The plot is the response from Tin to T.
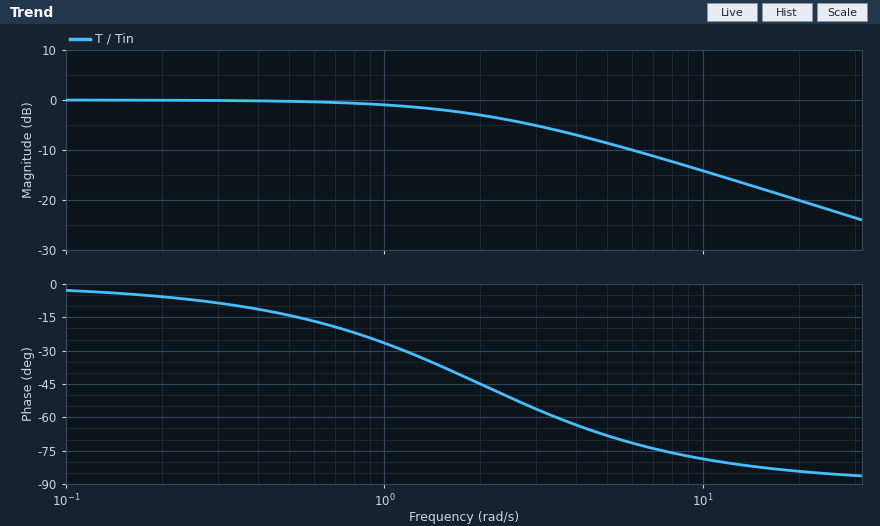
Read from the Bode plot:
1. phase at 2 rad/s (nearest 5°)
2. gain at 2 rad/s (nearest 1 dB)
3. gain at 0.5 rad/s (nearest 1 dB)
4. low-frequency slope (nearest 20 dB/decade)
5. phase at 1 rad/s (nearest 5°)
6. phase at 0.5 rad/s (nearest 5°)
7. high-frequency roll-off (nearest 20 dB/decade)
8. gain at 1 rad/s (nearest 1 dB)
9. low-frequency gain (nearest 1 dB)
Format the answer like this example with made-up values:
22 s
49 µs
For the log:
-45°
-3 dB
0 dB
0 dB/decade
-25°
-15°
-20 dB/decade
-1 dB
0 dB
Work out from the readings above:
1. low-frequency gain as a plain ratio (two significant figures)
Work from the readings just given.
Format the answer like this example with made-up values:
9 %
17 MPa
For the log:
1.0
